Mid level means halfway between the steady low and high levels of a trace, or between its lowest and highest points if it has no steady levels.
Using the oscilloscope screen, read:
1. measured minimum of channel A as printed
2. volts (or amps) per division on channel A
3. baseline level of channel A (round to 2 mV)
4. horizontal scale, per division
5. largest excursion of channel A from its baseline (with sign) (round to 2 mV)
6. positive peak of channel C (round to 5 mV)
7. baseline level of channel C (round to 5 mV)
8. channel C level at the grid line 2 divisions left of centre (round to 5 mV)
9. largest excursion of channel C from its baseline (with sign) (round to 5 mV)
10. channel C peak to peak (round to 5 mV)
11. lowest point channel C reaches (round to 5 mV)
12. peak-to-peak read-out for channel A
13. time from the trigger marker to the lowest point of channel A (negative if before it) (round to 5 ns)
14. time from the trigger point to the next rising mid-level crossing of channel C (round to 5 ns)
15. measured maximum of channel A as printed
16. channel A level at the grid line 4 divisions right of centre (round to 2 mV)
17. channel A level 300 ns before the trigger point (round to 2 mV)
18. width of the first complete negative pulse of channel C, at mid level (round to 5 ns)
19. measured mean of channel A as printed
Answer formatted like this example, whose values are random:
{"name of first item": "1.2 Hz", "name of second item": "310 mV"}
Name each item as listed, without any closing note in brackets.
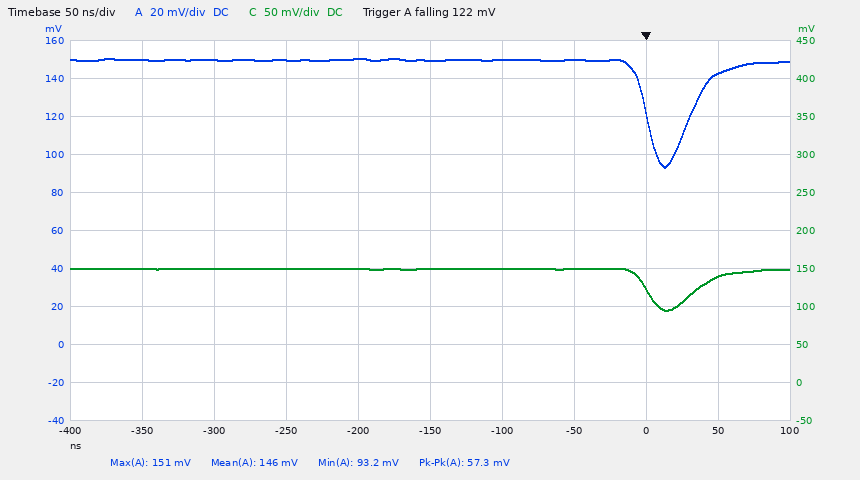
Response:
{"measured minimum of channel A as printed": "93.2 mV", "volts (or amps) per division on channel A": "20 mV", "baseline level of channel A": "150 mV", "horizontal scale, per division": "50 ns", "largest excursion of channel A from its baseline (with sign)": "-56 mV", "positive peak of channel C": "150 mV", "baseline level of channel C": "150 mV", "channel C level at the grid line 2 divisions left of centre": "150 mV", "largest excursion of channel C from its baseline (with sign)": "-55 mV", "channel C peak to peak": "55 mV", "lowest point channel C reaches": "95 mV", "peak-to-peak read-out for channel A": "57.3 mV", "time from the trigger marker to the lowest point of channel A (negative if before it)": "+15 ns", "time from the trigger point to the next rising mid-level crossing of channel C": "35 ns", "measured maximum of channel A as printed": "151 mV", "channel A level at the grid line 4 divisions right of centre": "142 mV", "channel A level 300 ns before the trigger point": "150 mV", "width of the first complete negative pulse of channel C, at mid level": "35 ns", "measured mean of channel A as printed": "146 mV"}
